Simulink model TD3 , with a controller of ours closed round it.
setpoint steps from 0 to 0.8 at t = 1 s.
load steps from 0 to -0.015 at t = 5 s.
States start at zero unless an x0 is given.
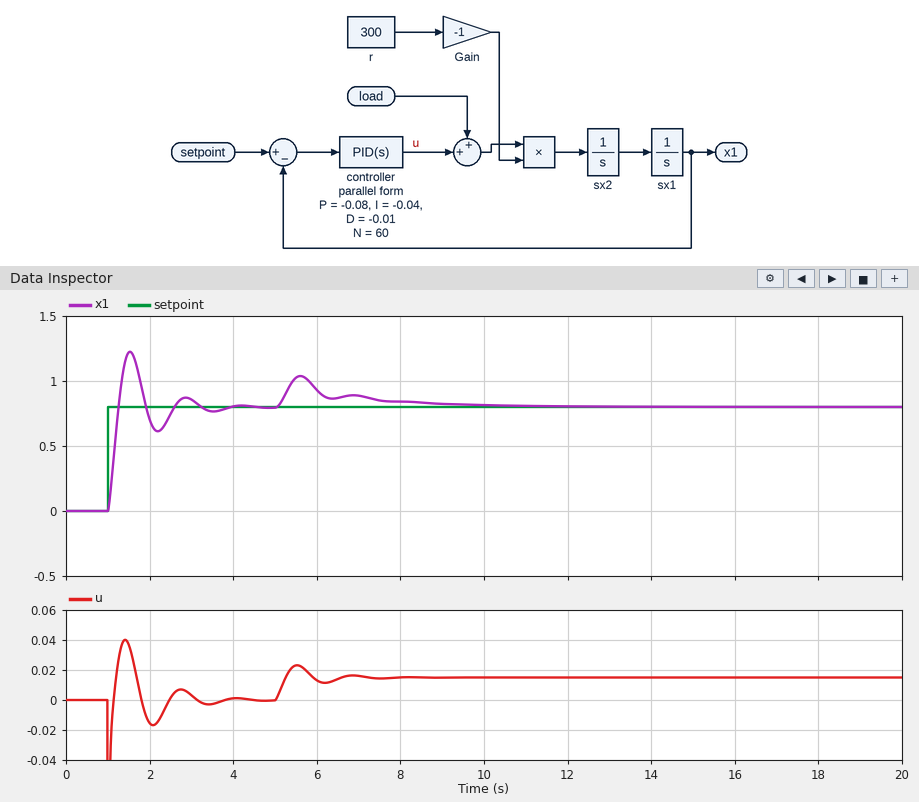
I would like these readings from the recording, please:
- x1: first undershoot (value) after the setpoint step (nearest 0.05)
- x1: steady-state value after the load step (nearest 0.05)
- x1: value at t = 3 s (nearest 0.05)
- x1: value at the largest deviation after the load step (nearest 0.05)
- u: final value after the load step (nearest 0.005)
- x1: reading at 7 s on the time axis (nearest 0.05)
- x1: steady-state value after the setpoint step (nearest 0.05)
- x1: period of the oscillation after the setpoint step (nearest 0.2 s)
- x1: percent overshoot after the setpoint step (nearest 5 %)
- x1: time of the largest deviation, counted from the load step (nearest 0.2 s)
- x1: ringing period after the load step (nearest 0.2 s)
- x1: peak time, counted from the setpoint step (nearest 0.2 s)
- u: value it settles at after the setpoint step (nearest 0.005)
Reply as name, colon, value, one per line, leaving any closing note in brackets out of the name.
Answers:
x1: first undershoot (value) after the setpoint step: 0.60
x1: steady-state value after the load step: 0.80
x1: value at t = 3 s: 0.85
x1: value at the largest deviation after the load step: 1.05
u: final value after the load step: 0.015
x1: reading at 7 s on the time axis: 0.90
x1: steady-state value after the setpoint step: 0.80
x1: period of the oscillation after the setpoint step: 1.4 s
x1: percent overshoot after the setpoint step: 55 %
x1: time of the largest deviation, counted from the load step: 0.6 s
x1: ringing period after the load step: 1.2 s
x1: peak time, counted from the setpoint step: 0.6 s
u: value it settles at after the setpoint step: 0.000
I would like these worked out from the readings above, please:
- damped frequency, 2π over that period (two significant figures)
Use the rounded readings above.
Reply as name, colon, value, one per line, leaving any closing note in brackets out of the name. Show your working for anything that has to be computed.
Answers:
damped frequency, 2π over that period: 2π / 1.4 = 4.5 rad/s
